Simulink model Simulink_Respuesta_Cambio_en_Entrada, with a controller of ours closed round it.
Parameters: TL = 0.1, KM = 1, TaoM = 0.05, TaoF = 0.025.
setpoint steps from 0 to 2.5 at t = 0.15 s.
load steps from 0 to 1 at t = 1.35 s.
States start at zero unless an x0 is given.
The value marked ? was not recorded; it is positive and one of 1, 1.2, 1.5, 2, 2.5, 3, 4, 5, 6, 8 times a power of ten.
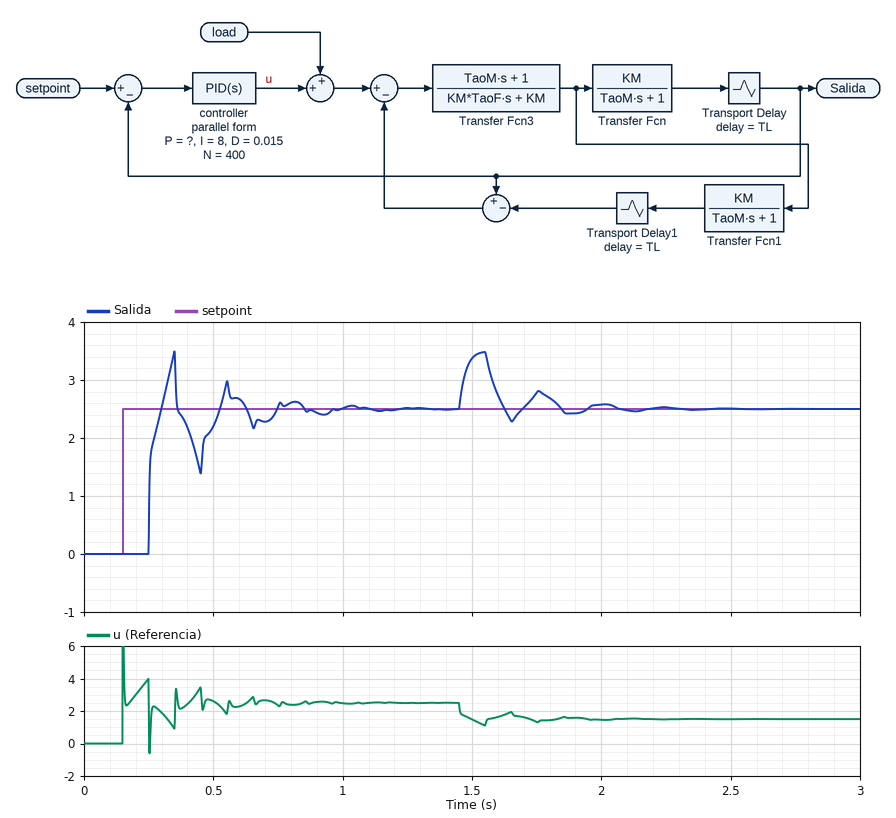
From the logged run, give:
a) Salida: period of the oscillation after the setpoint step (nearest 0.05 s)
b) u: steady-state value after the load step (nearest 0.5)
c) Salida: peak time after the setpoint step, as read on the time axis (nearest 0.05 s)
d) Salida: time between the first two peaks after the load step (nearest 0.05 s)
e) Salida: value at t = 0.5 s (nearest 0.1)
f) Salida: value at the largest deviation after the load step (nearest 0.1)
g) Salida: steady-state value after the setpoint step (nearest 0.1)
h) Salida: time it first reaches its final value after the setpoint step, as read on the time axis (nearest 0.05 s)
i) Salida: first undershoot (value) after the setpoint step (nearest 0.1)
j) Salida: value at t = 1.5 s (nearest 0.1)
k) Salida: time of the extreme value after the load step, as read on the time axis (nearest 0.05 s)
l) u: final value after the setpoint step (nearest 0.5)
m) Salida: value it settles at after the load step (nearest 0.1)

0.20 s
1.5
0.35 s
0.20 s
2.2
3.5
2.5
0.30 s
1.4
3.4
1.55 s
2.5
2.5
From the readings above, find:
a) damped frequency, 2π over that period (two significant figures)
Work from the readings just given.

31 rad/s
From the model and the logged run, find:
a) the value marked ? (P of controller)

0.8
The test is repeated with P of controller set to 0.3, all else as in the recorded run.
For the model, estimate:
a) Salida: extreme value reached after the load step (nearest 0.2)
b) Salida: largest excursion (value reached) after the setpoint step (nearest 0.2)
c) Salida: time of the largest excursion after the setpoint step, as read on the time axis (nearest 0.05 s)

3.4
3.0
0.45 s
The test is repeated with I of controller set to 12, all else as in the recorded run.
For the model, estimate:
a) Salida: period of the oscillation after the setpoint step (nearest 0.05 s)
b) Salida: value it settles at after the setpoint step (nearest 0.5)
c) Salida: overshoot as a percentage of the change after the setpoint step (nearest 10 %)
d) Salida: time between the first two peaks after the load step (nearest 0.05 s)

0.25 s
2.5
70 %
0.25 s
